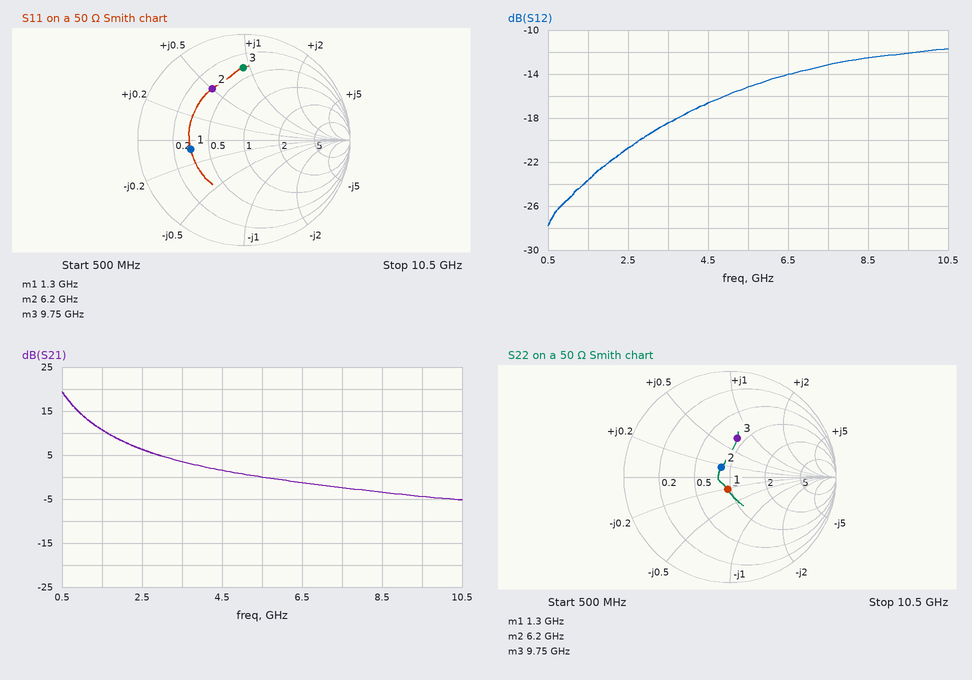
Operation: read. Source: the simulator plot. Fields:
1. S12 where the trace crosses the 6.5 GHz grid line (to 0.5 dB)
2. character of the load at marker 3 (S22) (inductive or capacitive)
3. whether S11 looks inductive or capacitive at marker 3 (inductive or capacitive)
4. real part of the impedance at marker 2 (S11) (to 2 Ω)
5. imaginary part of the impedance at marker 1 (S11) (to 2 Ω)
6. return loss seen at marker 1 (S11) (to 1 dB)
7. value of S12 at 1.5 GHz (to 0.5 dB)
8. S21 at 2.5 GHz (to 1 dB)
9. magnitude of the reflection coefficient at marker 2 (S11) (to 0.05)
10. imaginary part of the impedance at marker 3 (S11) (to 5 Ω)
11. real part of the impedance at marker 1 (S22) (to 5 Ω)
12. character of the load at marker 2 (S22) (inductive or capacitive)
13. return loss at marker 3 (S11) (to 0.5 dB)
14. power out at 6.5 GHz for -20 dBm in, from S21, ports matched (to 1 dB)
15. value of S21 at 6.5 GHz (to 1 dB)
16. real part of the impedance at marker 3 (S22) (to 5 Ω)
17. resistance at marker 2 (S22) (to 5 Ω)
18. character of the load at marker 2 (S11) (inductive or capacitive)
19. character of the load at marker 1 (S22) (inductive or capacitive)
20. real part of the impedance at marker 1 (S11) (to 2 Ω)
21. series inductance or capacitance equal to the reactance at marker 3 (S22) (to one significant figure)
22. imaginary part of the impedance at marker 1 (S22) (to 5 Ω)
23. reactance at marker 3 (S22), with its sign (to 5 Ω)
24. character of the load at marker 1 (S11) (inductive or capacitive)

-14.0 dB
inductive
inductive
18 Ω
-4 Ω
6 dB
-23.5 dB
6 dB
0.55
+45 Ω
45 Ω
inductive
3.5 dB
-21 dBm
-1 dB
45 Ω
40 Ω
inductive
capacitive
16 Ω
600 pH
-10 Ω
+35 Ω
capacitive
